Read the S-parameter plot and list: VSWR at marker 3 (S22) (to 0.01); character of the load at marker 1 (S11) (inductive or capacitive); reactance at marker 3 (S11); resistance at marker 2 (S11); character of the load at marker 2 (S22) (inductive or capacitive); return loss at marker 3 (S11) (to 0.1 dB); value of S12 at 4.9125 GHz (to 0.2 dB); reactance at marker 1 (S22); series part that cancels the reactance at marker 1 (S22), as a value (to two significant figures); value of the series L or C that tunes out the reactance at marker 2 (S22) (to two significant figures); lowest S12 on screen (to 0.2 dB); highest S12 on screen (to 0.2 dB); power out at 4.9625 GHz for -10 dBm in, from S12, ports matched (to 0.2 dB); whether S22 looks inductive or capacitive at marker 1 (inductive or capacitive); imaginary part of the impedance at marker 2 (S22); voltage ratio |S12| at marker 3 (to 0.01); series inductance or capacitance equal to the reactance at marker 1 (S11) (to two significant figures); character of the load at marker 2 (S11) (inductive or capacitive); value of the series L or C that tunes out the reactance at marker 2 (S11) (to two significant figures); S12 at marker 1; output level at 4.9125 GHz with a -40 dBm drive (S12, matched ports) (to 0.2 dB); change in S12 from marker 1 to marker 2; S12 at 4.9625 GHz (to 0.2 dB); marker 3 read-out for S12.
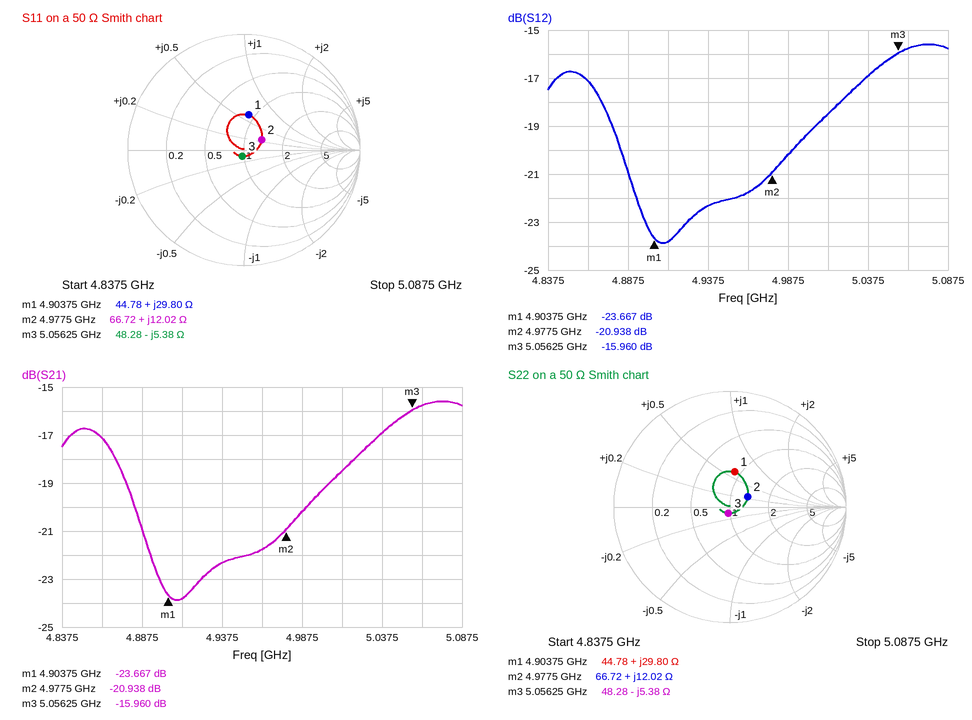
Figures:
1.12
inductive
-5.38 Ω
66.72 Ω
inductive
24.8 dB
-23.8 dB
+29.80 Ω
1.1 pF
2.7 pF
-23.8 dB
-15.6 dB
-31.8 dBm
inductive
+12.02 Ω
0.16
970 pH
inductive
2.7 pF
-23.667 dB
-63.8 dBm
2.729 dB
-21.8 dB
-15.960 dB
